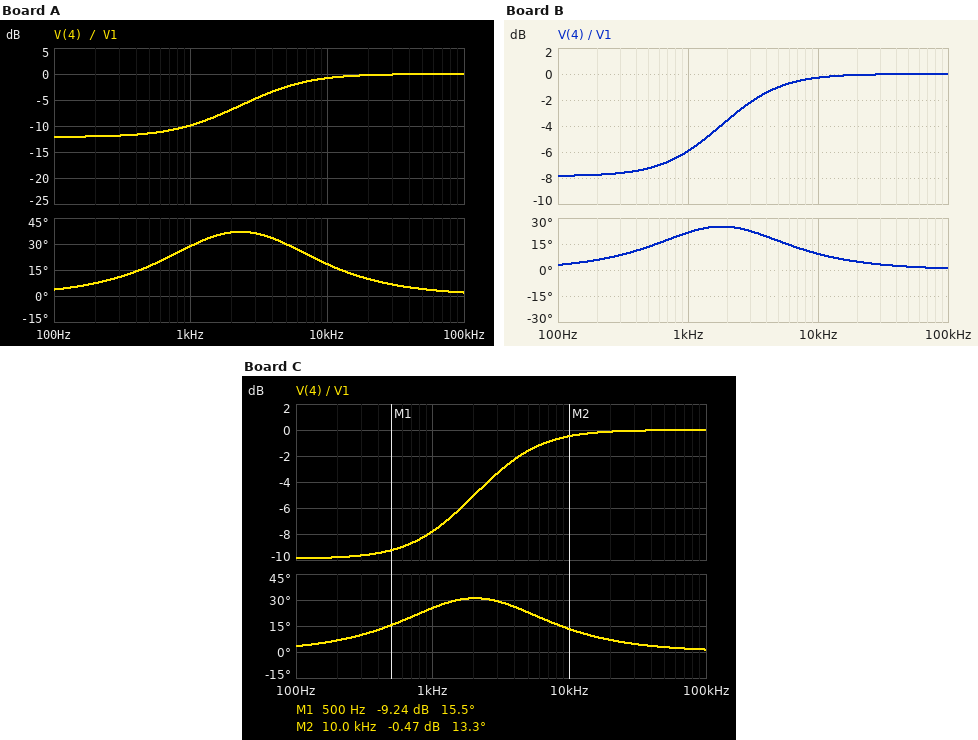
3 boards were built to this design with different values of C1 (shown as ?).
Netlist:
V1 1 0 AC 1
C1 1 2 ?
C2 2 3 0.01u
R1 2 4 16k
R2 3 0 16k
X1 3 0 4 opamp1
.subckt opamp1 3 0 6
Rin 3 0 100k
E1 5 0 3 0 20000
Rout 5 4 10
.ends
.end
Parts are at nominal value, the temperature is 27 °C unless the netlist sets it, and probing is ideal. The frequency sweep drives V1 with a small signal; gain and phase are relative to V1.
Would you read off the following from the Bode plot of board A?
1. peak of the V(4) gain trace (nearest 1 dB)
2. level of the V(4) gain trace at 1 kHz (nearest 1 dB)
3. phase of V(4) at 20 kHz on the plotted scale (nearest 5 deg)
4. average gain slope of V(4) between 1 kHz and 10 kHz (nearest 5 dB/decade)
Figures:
0 dB
-10 dB
10 deg
10 dB/decade
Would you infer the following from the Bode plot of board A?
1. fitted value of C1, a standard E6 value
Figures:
3.3 nF
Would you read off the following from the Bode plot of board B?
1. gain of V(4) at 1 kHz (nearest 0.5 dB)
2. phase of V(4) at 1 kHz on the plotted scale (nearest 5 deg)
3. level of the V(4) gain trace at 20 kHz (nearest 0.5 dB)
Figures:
-6.0 dB
20 deg
0 dB
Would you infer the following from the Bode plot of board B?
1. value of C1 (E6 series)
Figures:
6.8 nF
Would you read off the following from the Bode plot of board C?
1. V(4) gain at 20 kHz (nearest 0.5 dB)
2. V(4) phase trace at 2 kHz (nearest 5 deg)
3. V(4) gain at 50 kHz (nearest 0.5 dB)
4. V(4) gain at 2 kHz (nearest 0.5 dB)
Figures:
0 dB
30 deg
0 dB
-5.0 dB
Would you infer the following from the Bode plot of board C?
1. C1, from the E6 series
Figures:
4.7 nF
